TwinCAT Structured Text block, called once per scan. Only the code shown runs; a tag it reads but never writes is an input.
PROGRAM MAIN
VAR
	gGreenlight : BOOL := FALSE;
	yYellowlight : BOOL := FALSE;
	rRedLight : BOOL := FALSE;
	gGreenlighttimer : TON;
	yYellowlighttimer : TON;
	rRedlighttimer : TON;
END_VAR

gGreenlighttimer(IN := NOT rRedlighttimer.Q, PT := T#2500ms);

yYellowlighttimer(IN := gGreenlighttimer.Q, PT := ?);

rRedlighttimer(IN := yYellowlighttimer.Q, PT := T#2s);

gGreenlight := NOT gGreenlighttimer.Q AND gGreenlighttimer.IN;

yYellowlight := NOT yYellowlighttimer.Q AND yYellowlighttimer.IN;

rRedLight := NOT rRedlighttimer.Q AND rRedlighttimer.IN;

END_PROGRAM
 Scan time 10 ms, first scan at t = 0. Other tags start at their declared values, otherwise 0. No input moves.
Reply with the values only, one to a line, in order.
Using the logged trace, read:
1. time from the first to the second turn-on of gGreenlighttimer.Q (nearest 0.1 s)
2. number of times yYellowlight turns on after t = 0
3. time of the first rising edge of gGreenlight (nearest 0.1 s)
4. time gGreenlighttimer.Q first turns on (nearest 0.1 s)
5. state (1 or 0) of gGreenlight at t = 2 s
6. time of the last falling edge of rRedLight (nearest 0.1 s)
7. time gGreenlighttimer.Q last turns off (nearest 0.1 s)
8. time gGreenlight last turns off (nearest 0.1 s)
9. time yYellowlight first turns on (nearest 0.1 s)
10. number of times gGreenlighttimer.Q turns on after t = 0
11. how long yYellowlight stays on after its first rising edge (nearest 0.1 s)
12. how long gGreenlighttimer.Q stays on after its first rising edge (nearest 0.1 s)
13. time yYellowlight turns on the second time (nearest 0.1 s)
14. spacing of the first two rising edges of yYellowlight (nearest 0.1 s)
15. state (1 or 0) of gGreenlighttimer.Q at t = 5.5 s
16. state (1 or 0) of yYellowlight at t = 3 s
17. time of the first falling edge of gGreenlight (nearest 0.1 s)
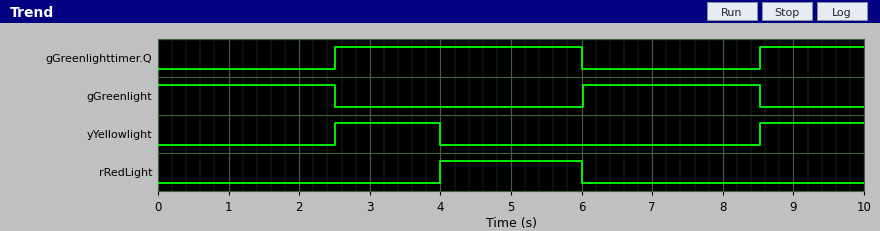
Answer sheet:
6.0 s
2
6.0 s
2.5 s
1
6.0 s
6.0 s
8.5 s
2.5 s
2
1.5 s
3.5 s
8.5 s
6.0 s
1
1
2.5 s
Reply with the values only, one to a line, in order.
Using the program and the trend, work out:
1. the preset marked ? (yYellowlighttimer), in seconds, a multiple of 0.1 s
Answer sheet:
1.5 s
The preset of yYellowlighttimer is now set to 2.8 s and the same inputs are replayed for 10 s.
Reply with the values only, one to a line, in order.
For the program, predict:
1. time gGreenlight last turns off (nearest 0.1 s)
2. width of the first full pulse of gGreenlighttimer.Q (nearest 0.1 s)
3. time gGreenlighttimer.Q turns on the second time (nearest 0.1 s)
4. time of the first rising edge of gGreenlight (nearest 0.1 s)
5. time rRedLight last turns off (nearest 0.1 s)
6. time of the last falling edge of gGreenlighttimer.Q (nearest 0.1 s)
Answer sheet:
9.8 s
4.8 s
9.8 s
7.3 s
7.3 s
7.3 s
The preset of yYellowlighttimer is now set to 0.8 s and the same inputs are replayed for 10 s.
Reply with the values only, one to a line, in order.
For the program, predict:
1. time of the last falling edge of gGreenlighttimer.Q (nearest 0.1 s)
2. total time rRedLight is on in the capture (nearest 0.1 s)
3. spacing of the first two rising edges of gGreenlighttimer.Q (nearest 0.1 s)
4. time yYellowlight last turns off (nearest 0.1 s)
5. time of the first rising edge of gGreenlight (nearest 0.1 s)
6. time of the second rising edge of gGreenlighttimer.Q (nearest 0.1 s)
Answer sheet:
5.3 s
3.4 s
5.3 s
8.6 s
5.3 s
7.8 s
